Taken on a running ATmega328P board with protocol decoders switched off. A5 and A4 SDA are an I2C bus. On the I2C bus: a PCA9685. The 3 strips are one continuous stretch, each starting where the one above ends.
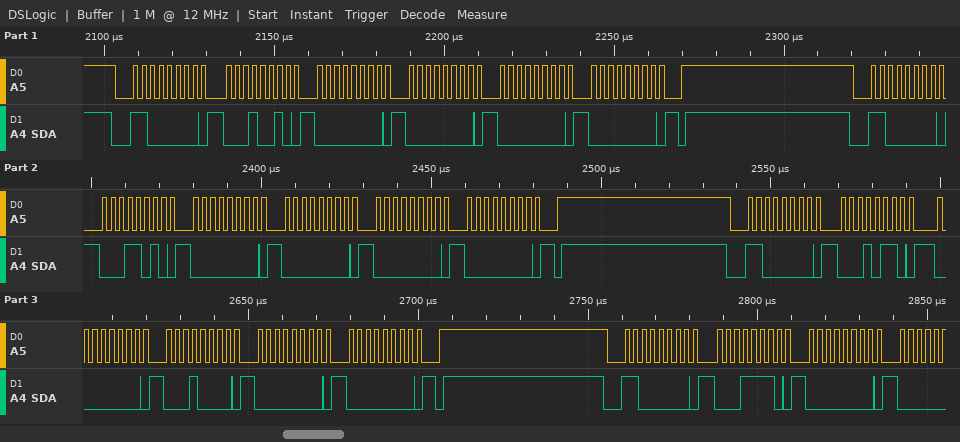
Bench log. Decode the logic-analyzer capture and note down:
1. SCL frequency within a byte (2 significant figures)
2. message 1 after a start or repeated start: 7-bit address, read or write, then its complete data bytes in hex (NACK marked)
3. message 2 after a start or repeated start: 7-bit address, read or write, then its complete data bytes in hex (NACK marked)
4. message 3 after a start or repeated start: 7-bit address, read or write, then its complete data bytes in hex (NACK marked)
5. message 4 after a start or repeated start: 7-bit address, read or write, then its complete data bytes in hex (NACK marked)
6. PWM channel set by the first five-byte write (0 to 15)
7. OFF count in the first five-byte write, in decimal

400 kHz
0x60 write: 12 00 00 00 00
0x60 write: 1A 00 00 00 00
0x60 write: 16 00 10 00 00
0x60 write: 1E 00
3
0
